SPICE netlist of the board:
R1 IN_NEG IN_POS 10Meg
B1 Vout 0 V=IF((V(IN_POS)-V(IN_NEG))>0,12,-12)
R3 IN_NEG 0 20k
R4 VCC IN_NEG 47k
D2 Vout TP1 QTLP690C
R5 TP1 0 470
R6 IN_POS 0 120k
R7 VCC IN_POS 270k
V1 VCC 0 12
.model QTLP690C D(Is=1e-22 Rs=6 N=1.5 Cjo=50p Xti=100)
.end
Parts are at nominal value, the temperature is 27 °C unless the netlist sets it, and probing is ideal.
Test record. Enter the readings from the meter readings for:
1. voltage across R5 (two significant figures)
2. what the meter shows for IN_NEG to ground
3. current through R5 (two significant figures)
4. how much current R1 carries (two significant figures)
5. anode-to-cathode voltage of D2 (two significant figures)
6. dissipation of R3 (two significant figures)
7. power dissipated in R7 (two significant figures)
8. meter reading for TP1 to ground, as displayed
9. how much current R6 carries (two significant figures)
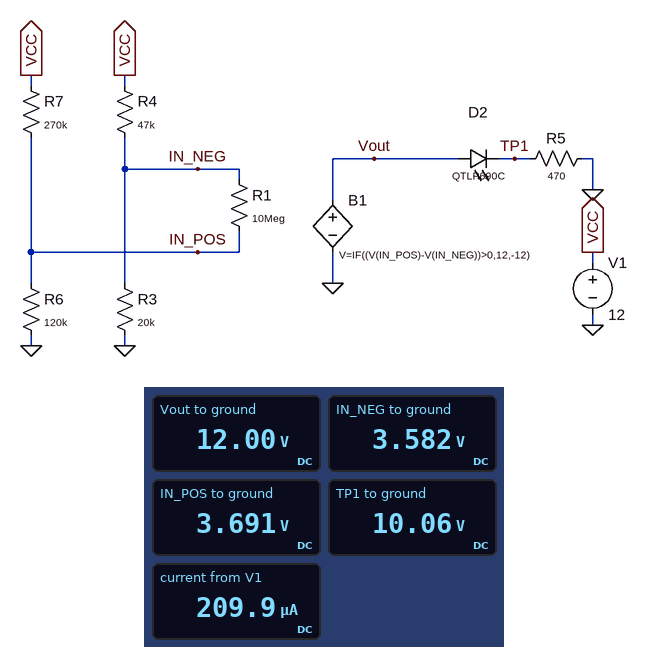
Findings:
10 V
3.582 V
21 mA
11 nA
1.9 V
640 µW
260 µW
10.06 V
31 µA
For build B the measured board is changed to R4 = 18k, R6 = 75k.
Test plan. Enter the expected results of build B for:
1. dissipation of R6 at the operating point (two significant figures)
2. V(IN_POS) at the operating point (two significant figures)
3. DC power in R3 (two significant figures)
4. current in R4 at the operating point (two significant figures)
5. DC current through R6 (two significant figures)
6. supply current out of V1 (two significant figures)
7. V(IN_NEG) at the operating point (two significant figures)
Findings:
92 µW
2.6 V
2.0 mW
320 µA
35 µA
350 µA
6.3 V
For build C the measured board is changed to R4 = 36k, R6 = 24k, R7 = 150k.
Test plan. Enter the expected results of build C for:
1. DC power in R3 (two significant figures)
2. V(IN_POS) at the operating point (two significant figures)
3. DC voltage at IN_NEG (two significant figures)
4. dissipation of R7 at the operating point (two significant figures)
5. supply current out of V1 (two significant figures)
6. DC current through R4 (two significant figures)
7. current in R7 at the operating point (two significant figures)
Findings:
920 µW
1.7 V
4.3 V
710 µW
280 µA
210 µA
69 µA
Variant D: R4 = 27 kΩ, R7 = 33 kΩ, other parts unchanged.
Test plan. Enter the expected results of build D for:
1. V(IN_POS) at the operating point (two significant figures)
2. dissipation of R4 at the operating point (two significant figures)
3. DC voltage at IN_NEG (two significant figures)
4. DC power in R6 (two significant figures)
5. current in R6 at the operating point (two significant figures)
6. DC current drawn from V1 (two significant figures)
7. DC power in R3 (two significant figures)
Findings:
9.4 V
1.8 mW
5.1 V
740 µW
78 µA
330 µA
1.3 mW
